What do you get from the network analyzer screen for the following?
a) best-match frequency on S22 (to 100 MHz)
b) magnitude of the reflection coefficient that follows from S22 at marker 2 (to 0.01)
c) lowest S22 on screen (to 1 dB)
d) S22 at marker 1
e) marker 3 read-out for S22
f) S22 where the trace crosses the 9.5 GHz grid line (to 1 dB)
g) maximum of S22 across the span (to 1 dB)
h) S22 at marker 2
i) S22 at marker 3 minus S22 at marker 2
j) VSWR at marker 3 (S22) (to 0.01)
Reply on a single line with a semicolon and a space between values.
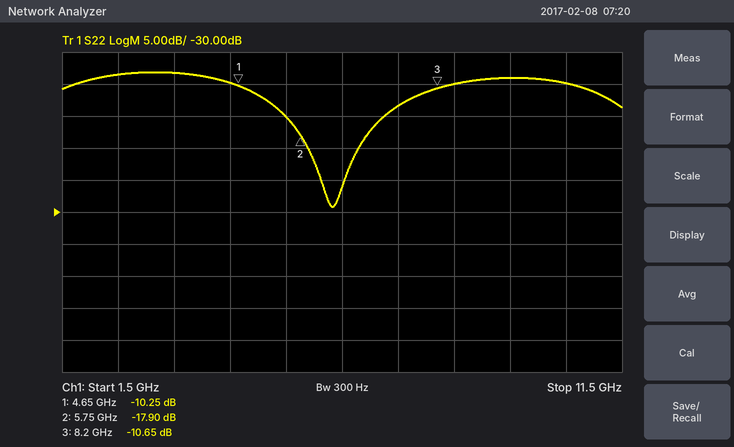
6.3 GHz; 0.13; -29 dB; -10.25 dB; -10.65 dB; -9 dB; -8 dB; -17.90 dB; 7.25 dB; 1.83
